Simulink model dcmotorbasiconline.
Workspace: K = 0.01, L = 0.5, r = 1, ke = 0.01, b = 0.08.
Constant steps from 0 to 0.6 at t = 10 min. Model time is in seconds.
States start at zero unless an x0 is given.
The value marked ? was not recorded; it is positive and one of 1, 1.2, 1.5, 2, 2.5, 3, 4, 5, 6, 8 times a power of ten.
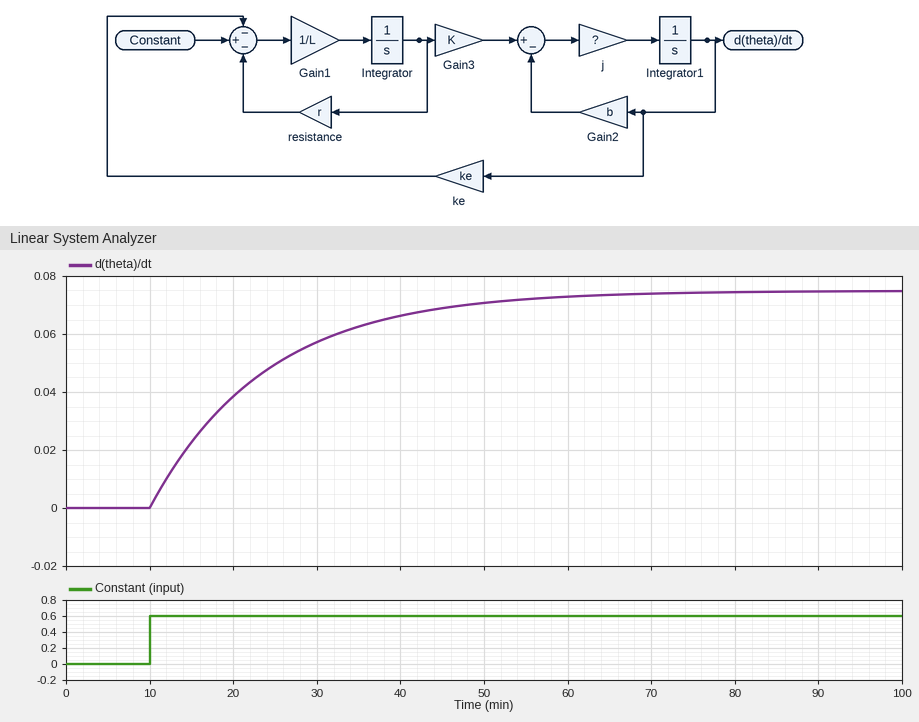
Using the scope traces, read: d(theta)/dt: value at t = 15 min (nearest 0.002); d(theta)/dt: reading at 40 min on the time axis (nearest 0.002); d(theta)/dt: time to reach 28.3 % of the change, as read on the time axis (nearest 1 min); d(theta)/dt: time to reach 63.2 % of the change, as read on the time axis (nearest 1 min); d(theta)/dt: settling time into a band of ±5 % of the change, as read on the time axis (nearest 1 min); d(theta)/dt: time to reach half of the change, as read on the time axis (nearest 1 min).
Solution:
0.022
0.066
15 min
24 min
52 min
20 min
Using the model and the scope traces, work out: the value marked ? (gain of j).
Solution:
0.015
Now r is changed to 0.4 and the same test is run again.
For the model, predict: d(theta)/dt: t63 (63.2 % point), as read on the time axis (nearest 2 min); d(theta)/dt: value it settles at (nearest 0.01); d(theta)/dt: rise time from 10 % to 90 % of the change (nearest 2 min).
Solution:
24 min
0.19
30 min
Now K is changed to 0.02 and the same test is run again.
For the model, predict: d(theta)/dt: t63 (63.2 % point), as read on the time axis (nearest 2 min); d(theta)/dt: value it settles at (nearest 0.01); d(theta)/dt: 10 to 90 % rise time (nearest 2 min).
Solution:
24 min
0.15
30 min
